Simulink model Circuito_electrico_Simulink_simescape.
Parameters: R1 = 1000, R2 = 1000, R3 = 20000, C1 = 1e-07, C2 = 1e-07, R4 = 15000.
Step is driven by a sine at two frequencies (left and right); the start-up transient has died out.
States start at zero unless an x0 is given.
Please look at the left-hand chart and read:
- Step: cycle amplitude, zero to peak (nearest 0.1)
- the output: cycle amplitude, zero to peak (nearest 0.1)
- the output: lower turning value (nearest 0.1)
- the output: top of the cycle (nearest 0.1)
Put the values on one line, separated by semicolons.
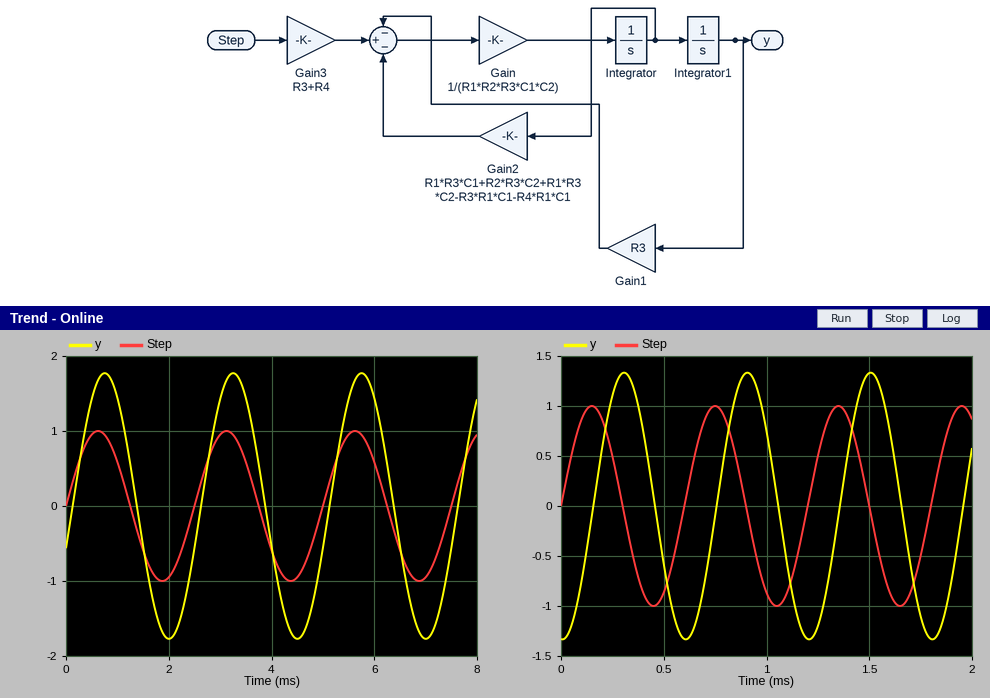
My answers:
1.0; 1.8; -1.8; 1.8
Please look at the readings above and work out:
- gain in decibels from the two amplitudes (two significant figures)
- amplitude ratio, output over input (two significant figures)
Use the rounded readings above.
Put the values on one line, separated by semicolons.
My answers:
5.1 dB; 1.8
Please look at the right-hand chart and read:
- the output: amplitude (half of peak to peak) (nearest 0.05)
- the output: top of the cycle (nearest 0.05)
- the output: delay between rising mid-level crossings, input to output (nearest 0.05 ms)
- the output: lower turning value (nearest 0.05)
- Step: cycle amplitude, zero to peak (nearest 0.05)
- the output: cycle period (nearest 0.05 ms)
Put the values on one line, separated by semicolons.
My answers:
1.35; 1.35; 0.15 ms; -1.35; 1.00; 0.60 ms
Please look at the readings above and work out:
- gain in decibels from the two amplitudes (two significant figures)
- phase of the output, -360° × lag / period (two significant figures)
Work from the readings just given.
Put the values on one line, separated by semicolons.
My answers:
2.6 dB; -90°
